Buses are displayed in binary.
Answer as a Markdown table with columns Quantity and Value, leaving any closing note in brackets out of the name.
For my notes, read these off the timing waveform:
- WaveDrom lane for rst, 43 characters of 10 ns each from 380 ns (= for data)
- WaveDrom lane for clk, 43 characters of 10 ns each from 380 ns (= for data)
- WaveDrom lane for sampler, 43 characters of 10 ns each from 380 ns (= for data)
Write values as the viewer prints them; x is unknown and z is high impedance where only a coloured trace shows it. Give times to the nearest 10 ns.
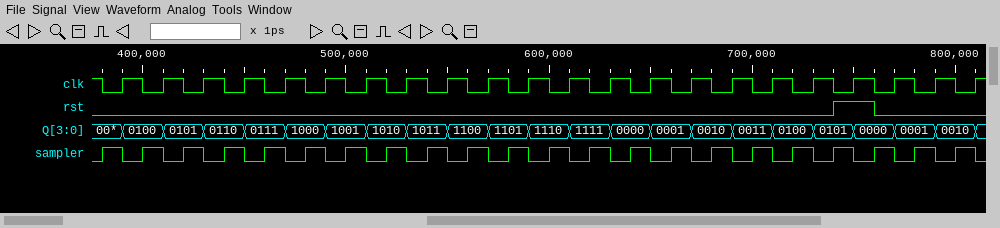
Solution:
| Quantity | Value |
|---|---|
| WaveDrom lane for rst, 43 characters of 10 ns each from 380 ns | {name: 'rst', wave: '0...................................1.0....'} |
| WaveDrom lane for clk, 43 characters of 10 ns each from 380 ns | {name: 'clk', wave: '0101010101010101010101010101010101010101010'} |
| WaveDrom lane for sampler, 43 characters of 10 ns each from 380 ns | {name: 'sampler', wave: '1010101010101010101010101010101010101010101'} |
